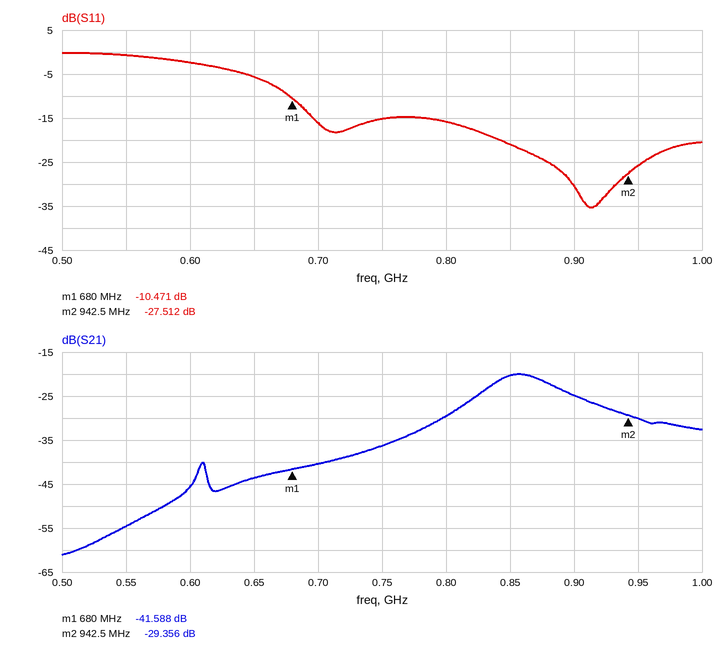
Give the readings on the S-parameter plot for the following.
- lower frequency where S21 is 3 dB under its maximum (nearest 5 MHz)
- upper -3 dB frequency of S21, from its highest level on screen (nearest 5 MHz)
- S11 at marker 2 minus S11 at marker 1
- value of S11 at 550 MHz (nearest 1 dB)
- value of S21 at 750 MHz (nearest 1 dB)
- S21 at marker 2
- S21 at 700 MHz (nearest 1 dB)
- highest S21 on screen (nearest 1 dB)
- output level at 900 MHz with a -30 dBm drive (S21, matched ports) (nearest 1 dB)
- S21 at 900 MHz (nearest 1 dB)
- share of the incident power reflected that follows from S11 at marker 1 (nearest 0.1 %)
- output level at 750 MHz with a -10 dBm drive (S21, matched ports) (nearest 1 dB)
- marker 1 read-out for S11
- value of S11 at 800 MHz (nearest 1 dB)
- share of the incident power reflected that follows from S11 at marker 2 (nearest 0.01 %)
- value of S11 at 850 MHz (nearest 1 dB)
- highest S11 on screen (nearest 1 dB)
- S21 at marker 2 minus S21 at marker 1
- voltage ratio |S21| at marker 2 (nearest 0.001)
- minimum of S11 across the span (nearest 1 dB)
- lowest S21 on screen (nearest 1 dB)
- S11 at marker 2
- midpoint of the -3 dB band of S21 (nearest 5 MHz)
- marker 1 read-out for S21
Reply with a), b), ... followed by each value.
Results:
a) 835 MHz
b) 885 MHz
c) -17.041 dB
d) -1 dB
e) -36 dB
f) -29.356 dB
g) -40 dB
h) -20 dB
i) -55 dBm
j) -25 dB
k) 9.0 %
l) -46 dBm
m) -10.471 dB
n) -16 dB
o) 0.18 %
p) -21 dB
q) 0 dB
r) 12.232 dB
s) 0.034
t) -35 dB
u) -61 dB
v) -27.512 dB
w) 860 MHz
x) -41.588 dB
